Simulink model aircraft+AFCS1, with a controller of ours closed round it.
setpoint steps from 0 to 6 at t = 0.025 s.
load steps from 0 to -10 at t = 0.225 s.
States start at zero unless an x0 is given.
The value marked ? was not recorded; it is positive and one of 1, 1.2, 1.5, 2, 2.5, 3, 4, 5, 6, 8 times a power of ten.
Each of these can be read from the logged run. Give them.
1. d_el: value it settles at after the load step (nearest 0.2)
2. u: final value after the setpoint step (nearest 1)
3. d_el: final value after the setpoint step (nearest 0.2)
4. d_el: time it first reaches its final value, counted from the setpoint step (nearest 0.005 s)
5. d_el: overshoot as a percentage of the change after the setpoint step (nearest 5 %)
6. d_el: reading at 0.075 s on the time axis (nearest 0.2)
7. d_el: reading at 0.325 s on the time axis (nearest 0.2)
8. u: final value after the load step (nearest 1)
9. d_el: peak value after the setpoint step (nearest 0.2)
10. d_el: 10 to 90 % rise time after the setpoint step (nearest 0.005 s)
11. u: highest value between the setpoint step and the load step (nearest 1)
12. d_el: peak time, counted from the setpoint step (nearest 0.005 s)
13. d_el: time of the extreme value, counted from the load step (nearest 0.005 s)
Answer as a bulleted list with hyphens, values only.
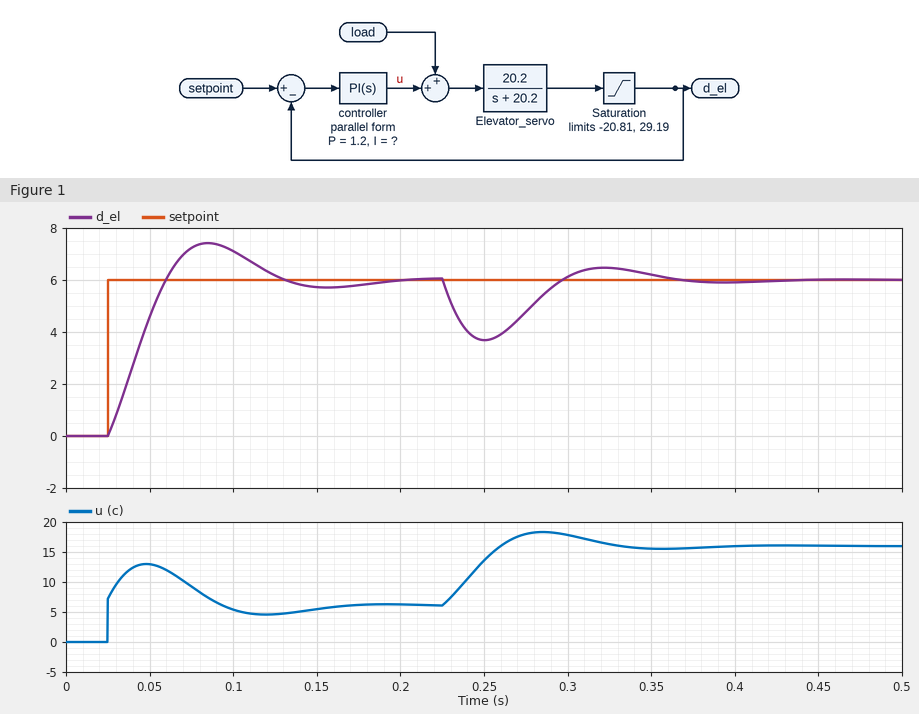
- 6.0
- 6
- 6.0
- 0.035 s
- 25 %
- 7.2
- 6.4
- 16
- 7.4
- 0.025 s
- 13
- 0.060 s
- 0.025 s
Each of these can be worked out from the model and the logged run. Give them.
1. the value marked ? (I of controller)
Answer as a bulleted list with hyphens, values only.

- 120
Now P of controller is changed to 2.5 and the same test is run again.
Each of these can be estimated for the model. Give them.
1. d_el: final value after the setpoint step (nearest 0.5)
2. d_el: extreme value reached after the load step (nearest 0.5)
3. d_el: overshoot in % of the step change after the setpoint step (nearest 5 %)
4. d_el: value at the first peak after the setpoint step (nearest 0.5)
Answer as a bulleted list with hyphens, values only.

- 6.0
- 4.0
- 10 %
- 6.5
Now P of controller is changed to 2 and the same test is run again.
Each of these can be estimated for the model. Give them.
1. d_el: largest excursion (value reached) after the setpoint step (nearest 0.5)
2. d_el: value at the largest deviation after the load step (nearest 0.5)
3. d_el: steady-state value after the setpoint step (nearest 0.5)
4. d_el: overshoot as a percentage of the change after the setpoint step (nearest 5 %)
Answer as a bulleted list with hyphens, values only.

- 7.0
- 4.0
- 6.0
- 15 %
